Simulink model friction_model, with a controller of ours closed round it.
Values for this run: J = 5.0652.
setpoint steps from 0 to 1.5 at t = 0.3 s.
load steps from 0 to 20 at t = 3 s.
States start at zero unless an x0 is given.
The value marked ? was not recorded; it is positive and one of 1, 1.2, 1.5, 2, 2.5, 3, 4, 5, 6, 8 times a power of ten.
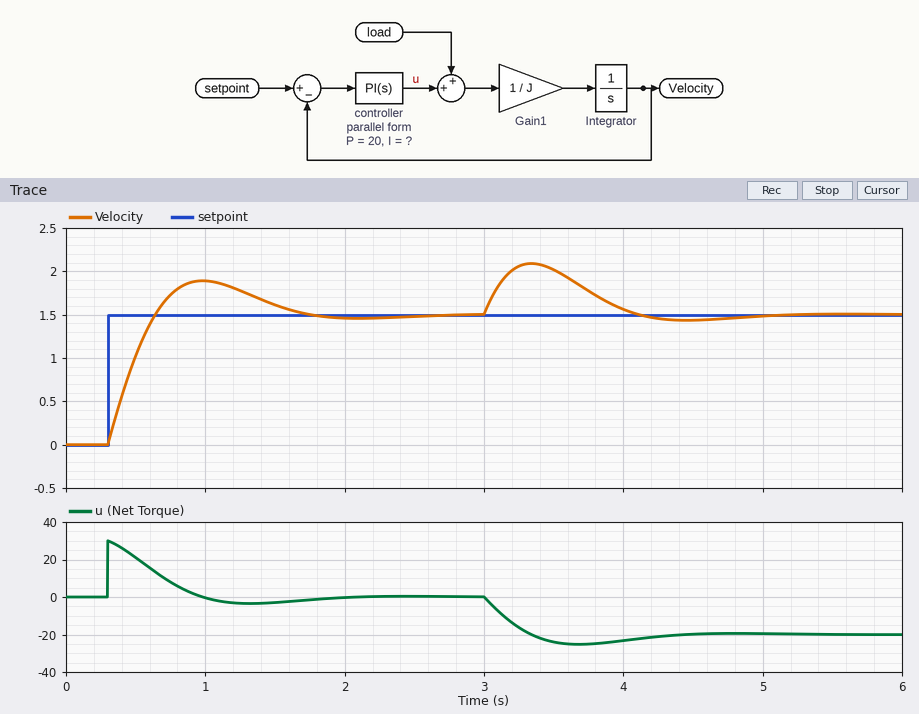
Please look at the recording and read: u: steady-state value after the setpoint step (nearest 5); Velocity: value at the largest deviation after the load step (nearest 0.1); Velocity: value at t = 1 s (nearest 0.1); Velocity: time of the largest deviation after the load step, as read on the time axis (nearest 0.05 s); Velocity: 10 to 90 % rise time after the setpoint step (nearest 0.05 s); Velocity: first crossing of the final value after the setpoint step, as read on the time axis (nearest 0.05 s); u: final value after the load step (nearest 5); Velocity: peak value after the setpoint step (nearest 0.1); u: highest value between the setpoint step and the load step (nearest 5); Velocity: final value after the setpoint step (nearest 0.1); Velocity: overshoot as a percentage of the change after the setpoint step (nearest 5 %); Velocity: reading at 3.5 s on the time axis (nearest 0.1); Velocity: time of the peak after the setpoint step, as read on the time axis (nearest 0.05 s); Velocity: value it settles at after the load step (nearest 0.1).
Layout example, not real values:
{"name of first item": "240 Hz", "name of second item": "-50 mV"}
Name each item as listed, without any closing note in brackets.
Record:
{"u: steady-state value after the setpoint step": "0", "Velocity: value at the largest deviation after the load step": "2.1", "Velocity: value at t = 1 s": "1.9", "Velocity: time of the largest deviation after the load step, as read on the time axis": "3.35 s", "Velocity: 10 to 90 % rise time after the setpoint step": "0.25 s", "Velocity: first crossing of the final value after the setpoint step, as read on the time axis": "0.65 s", "u: final value after the load step": "-20", "Velocity: peak value after the setpoint step": "1.9", "u: highest value between the setpoint step and the load step": "30", "Velocity: final value after the setpoint step": "1.5", "Velocity: overshoot as a percentage of the change after the setpoint step": "25 %", "Velocity: reading at 3.5 s on the time axis": "2.0", "Velocity: time of the peak after the setpoint step, as read on the time axis": "1.00 s", "Velocity: value it settles at after the load step": "1.5"}
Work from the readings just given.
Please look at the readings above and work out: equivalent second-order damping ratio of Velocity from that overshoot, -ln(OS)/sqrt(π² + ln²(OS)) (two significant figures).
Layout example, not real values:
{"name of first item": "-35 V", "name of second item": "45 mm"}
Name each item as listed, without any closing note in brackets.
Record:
{"equivalent second-order damping ratio of Velocity from that overshoot, -ln(OS)/sqrt(π² + ln²(OS))": "0.40"}
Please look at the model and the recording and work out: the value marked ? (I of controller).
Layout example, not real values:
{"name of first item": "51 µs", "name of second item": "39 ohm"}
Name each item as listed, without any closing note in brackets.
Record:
{"the value marked ?": "60"}
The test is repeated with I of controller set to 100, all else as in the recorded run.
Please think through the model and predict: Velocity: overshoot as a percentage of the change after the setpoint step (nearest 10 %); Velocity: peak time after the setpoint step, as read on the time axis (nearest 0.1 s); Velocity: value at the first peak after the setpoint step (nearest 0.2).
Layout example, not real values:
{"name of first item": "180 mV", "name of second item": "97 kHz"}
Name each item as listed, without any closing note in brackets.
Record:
{"Velocity: overshoot as a percentage of the change after the setpoint step": "30 %", "Velocity: peak time after the setpoint step, as read on the time axis": "0.9 s", "Velocity: value at the first peak after the setpoint step": "2.0"}
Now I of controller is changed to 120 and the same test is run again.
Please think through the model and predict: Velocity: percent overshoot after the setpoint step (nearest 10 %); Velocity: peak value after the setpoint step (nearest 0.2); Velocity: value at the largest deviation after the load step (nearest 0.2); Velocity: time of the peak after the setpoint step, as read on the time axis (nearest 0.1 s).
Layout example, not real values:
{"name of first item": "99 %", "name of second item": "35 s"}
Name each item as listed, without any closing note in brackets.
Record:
{"Velocity: percent overshoot after the setpoint step": "40 %", "Velocity: peak value after the setpoint step": "2.0", "Velocity: value at the largest deviation after the load step": "2.0", "Velocity: time of the peak after the setpoint step, as read on the time axis": "0.8 s"}
